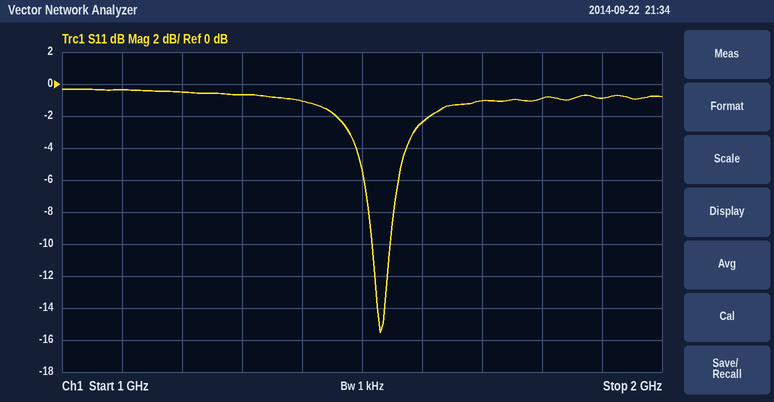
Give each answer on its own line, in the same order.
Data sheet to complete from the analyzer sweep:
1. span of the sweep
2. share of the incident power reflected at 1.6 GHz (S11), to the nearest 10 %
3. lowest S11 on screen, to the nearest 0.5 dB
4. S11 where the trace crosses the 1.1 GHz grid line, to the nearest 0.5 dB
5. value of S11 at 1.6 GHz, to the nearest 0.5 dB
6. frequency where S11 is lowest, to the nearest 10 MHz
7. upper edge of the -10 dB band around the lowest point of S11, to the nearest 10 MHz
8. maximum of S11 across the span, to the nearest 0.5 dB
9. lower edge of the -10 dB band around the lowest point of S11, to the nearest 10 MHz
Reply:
1 GHz
60 %
-15.5 dB
-0.5 dB
-2.5 dB
1.53 GHz
1.55 GHz
-0.5 dB
1.52 GHz
